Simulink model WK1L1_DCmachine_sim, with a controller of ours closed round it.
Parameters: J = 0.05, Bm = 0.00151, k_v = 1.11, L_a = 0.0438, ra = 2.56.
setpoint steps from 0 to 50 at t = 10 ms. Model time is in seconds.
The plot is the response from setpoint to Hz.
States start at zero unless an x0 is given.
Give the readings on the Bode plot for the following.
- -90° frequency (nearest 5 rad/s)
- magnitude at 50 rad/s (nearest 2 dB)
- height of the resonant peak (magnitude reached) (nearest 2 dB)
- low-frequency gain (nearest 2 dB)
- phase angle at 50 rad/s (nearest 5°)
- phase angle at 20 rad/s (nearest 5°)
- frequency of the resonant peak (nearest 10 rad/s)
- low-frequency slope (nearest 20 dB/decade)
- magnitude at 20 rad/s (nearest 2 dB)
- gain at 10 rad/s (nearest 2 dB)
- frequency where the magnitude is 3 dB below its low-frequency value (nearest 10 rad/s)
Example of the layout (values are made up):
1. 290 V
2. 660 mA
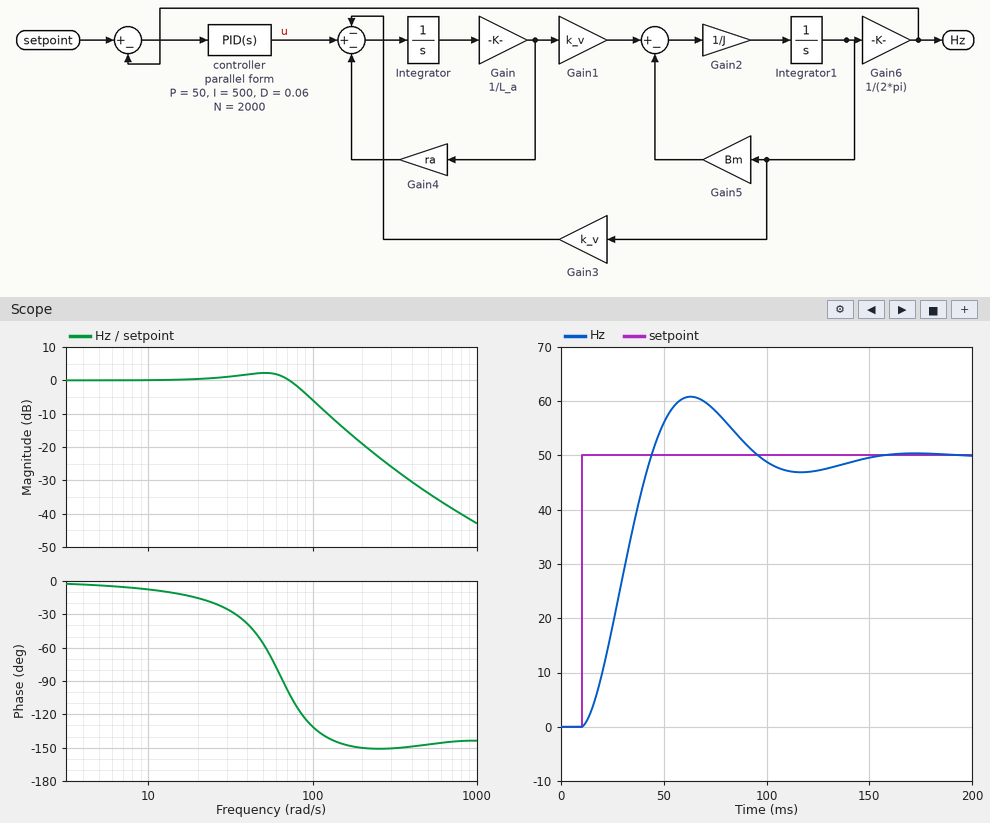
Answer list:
1. 65 rad/s
2. 2 dB
3. 2 dB
4. 0 dB
5. -55°
6. -15°
7. 50 rad/s
8. 0 dB/decade
9. 0 dB
10. 0 dB
11. 90 rad/s
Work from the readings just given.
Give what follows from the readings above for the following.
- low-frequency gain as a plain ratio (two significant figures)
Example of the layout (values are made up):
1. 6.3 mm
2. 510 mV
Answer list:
1. 1.0
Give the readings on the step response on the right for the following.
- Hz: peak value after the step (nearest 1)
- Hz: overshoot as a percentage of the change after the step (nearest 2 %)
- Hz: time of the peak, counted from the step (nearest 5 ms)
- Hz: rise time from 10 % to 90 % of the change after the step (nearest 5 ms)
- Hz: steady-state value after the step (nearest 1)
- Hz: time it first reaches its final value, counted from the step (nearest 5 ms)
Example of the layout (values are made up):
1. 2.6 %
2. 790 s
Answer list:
1. 61
2. 22 %
3. 55 ms
4. 25 ms
5. 50
6. 35 ms
